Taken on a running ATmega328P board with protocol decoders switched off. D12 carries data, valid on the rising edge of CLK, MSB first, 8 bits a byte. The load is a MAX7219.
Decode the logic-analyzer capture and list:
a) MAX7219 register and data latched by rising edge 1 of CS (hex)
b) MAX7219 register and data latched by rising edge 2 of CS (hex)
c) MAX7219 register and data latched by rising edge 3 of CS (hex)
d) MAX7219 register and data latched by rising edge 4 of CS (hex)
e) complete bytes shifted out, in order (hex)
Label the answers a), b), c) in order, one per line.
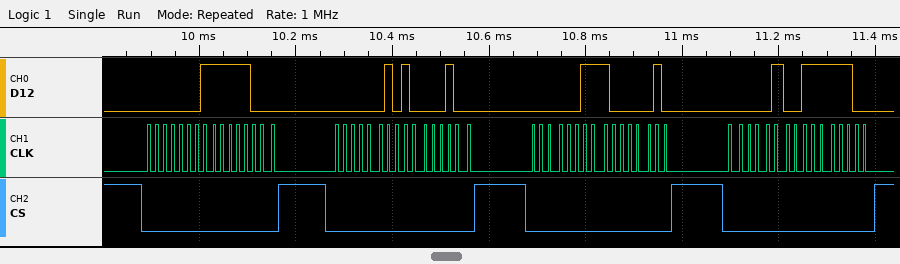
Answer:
a) register 0x1, data 0xF8
b) register 0x2, data 0x84
c) register 0x3, data 0x82
d) register 0x4, data 0xFC
e) 0x01 0xF8 0x02 0x84 0x03 0x82 0x04 0xFC
